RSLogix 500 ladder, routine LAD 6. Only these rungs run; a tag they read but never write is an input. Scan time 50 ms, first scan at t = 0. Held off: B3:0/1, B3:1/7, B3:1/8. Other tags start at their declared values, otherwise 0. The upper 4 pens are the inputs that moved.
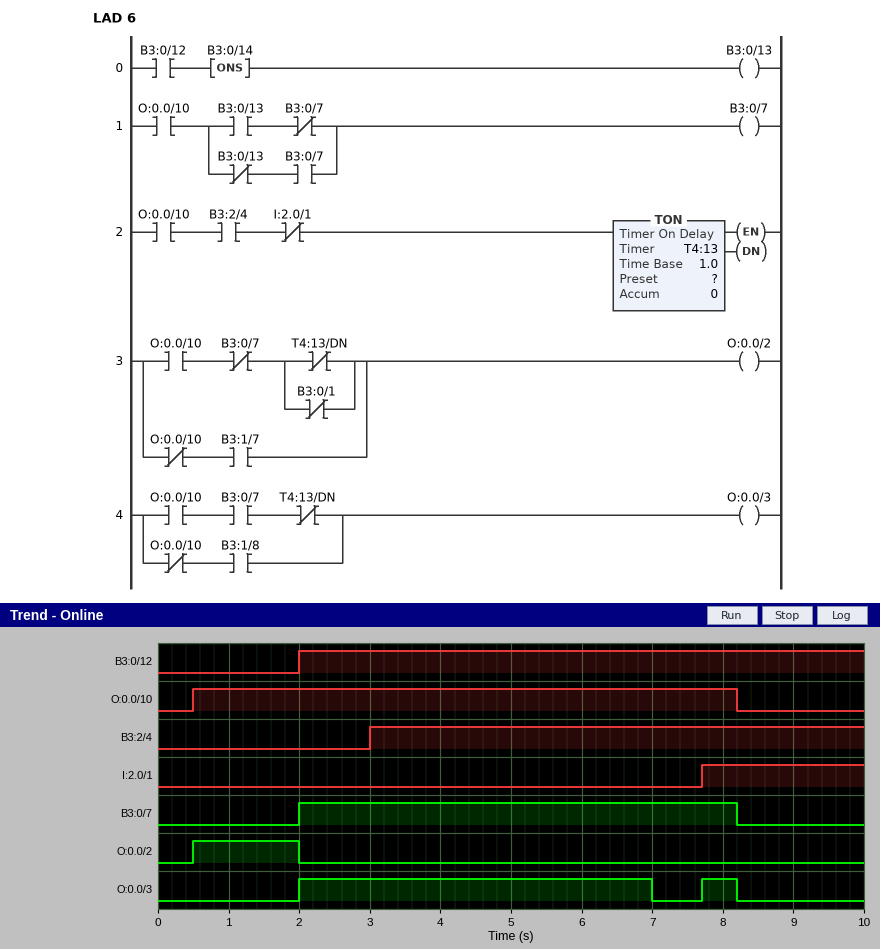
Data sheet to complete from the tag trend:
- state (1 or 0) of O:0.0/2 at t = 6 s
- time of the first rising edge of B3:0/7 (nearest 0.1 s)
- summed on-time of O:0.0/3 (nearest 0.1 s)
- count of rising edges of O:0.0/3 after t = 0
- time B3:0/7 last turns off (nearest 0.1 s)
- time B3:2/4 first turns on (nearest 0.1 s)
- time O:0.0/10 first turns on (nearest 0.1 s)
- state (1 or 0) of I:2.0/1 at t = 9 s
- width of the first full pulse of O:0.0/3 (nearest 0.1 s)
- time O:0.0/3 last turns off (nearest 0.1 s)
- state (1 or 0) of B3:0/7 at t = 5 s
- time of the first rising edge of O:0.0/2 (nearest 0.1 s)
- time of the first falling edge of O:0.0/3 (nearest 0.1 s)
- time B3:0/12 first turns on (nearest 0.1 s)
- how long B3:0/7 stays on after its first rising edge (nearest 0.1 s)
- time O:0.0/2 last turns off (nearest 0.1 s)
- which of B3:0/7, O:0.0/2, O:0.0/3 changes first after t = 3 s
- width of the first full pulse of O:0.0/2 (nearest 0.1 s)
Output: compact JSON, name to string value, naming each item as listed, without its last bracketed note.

{"state (1 or 0) of O:0.0/2 at t = 6 s": "0", "time of the first rising edge of B3:0/7": "2.0 s", "summed on-time of O:0.0/3": "5.5 s", "count of rising edges of O:0.0/3 after t = 0": "2", "time B3:0/7 last turns off": "8.2 s", "time B3:2/4 first turns on": "3.0 s", "time O:0.0/10 first turns on": "0.5 s", "state (1 or 0) of I:2.0/1 at t = 9 s": "1", "width of the first full pulse of O:0.0/3": "5.0 s", "time O:0.0/3 last turns off": "8.2 s", "state (1 or 0) of B3:0/7 at t = 5 s": "1", "time of the first rising edge of O:0.0/2": "0.5 s", "time of the first falling edge of O:0.0/3": "7.0 s", "time B3:0/12 first turns on": "2.0 s", "how long B3:0/7 stays on after its first rising edge": "6.2 s", "time O:0.0/2 last turns off": "2.0 s", "which of B3:0/7, O:0.0/2, O:0.0/3 changes first after t = 3 s": "O:0.0/3", "width of the first full pulse of O:0.0/2": "1.5 s"}
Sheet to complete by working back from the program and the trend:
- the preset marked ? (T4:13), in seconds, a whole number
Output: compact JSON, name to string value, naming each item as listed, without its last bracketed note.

{"the preset marked ? (T4:13), in seconds, a whole number": "4 s"}
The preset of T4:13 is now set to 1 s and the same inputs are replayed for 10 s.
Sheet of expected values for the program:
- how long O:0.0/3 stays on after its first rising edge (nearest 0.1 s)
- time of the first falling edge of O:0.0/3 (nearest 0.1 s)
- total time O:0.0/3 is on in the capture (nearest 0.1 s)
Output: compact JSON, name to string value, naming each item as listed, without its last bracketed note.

{"how long O:0.0/3 stays on after its first rising edge": "2.0 s", "time of the first falling edge of O:0.0/3": "4.0 s", "total time O:0.0/3 is on in the capture": "2.5 s"}
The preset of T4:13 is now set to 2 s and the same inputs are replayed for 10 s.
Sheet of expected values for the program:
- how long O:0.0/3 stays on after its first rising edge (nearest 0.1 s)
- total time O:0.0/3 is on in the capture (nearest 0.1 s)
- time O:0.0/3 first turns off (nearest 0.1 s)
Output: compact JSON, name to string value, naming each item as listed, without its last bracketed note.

{"how long O:0.0/3 stays on after its first rising edge": "3.0 s", "total time O:0.0/3 is on in the capture": "3.5 s", "time O:0.0/3 first turns off": "5.0 s"}
